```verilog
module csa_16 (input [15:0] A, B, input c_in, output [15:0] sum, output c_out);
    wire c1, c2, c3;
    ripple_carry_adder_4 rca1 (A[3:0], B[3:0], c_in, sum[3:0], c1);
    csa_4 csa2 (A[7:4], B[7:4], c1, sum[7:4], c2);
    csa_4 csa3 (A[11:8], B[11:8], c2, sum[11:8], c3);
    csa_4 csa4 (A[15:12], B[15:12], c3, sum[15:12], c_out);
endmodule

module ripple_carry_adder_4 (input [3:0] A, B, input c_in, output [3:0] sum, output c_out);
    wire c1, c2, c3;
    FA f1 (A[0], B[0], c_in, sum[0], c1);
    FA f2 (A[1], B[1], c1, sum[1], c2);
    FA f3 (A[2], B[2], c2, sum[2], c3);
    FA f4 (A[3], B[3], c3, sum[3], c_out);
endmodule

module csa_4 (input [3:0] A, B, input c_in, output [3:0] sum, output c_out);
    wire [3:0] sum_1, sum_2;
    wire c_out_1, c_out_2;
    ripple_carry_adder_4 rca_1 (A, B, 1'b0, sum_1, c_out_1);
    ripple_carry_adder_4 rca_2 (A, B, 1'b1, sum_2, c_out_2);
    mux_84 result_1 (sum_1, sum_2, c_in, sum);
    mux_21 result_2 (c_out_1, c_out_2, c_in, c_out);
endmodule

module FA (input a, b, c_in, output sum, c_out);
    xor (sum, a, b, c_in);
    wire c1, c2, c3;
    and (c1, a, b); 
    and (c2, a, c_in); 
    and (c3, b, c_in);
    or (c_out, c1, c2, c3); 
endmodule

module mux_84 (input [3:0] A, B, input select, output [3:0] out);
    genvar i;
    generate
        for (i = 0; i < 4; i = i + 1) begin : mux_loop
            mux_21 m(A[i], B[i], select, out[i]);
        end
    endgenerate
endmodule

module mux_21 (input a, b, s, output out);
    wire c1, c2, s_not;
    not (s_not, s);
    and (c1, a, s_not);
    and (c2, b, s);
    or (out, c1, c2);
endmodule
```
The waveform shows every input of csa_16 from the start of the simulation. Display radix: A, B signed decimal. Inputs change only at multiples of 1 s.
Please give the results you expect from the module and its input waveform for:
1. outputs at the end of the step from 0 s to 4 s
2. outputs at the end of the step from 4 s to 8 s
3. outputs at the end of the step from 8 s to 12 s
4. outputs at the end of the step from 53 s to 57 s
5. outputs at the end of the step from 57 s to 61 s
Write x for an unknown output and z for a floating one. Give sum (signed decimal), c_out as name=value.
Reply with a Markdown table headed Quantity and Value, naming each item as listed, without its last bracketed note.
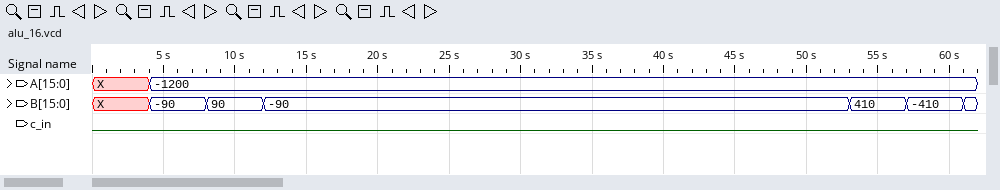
| Quantity | Value |
|---|---|
| outputs at the end of the step from 0 s to 4 s | sum=x, c_out=x |
| outputs at the end of the step from 4 s to 8 s | sum=-1290, c_out=1 |
| outputs at the end of the step from 8 s to 12 s | sum=-1110, c_out=0 |
| outputs at the end of the step from 53 s to 57 s | sum=-790, c_out=0 |
| outputs at the end of the step from 57 s to 61 s | sum=-1610, c_out=1 |
